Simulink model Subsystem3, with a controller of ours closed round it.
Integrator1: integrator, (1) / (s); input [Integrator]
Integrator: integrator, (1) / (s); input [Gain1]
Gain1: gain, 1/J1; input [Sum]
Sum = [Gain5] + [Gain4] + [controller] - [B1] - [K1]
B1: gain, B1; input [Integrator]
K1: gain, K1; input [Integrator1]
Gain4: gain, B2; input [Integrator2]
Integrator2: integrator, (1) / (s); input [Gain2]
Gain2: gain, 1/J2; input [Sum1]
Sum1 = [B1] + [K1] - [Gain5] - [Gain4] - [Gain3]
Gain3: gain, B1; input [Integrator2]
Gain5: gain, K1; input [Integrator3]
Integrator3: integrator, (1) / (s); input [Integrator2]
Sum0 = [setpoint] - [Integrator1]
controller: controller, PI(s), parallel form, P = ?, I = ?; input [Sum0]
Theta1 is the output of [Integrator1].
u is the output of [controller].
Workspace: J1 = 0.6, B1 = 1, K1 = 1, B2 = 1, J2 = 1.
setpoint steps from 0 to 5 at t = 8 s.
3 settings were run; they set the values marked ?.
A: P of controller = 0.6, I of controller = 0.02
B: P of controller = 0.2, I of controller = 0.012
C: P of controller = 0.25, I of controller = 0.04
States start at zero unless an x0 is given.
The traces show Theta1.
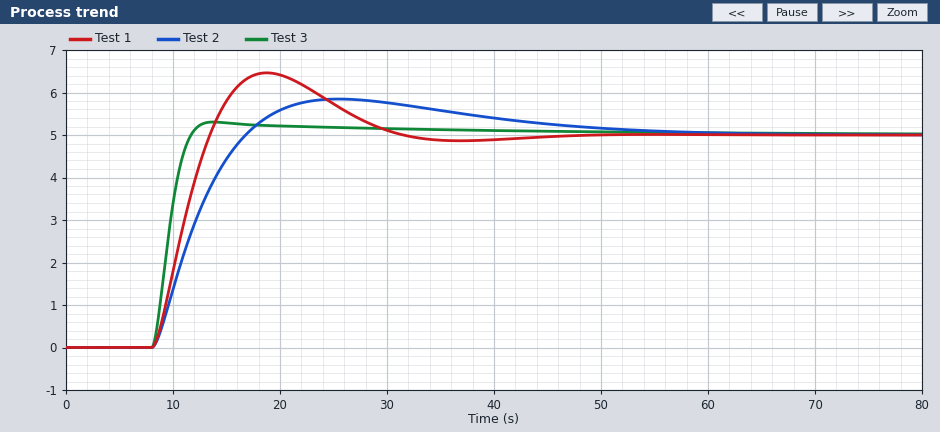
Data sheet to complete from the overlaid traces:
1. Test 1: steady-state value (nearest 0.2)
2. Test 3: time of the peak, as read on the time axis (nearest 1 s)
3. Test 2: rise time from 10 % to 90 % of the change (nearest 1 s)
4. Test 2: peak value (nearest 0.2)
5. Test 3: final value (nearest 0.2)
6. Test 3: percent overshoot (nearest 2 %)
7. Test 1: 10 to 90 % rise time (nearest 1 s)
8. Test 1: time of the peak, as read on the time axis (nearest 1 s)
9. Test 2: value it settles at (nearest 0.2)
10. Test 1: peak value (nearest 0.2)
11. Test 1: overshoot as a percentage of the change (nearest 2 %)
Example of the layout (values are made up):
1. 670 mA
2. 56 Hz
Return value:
1. 5.0
2. 14 s
3. 6 s
4. 5.8
5. 5.0
6. 6 %
7. 4 s
8. 19 s
9. 5.0
10. 6.4
11. 30 %
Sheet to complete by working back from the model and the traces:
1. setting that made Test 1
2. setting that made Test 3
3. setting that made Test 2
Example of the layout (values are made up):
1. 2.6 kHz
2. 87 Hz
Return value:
1. C
2. A
3. B
